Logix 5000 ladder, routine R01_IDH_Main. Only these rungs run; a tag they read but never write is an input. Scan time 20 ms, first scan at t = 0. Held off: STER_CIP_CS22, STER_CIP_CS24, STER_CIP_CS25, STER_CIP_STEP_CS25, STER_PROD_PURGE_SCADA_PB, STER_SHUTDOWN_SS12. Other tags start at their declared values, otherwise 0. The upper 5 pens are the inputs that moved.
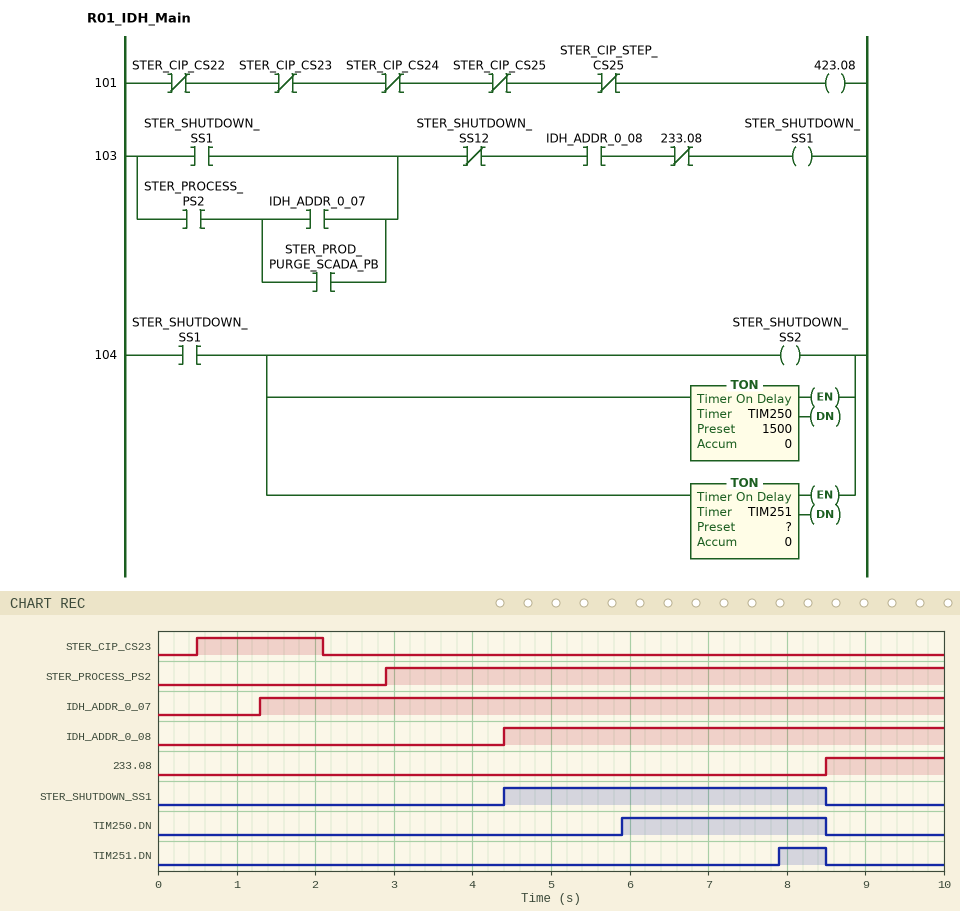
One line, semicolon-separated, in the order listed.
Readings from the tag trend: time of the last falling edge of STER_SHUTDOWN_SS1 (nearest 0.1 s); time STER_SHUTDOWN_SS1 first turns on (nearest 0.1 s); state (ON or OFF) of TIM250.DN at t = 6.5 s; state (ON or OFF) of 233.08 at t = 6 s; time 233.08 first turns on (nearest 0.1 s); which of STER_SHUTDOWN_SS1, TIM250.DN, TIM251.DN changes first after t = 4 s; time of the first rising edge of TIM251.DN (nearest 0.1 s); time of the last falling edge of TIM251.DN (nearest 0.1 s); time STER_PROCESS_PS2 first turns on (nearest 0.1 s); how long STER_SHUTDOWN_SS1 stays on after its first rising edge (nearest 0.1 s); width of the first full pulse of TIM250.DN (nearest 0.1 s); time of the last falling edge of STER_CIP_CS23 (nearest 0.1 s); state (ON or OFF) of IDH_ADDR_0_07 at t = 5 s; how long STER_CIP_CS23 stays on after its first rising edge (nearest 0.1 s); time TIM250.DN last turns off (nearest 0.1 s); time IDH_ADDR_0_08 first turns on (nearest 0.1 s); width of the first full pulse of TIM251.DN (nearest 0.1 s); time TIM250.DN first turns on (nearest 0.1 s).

8.5 s; 4.4 s; ON; OFF; 8.5 s; STER_SHUTDOWN_SS1; 7.9 s; 8.5 s; 2.9 s; 4.1 s; 2.6 s; 2.1 s; ON; 1.6 s; 8.5 s; 4.4 s; 0.6 s; 5.9 s
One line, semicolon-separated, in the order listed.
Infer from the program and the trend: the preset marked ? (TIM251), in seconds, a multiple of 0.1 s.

3.5 s
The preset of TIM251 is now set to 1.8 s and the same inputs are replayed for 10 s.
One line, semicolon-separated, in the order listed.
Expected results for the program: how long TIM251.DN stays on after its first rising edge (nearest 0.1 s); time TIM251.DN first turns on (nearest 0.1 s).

2.3 s; 6.2 s
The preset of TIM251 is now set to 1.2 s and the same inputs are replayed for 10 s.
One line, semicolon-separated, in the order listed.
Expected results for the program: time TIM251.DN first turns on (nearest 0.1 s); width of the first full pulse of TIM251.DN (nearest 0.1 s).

5.6 s; 2.9 s
